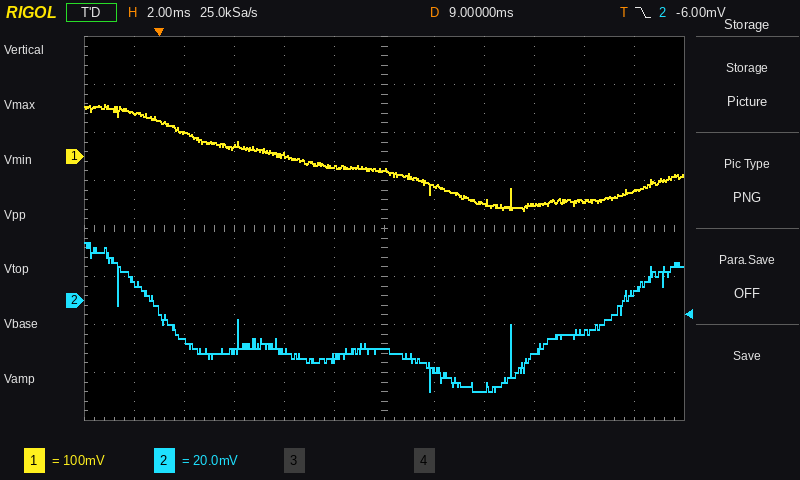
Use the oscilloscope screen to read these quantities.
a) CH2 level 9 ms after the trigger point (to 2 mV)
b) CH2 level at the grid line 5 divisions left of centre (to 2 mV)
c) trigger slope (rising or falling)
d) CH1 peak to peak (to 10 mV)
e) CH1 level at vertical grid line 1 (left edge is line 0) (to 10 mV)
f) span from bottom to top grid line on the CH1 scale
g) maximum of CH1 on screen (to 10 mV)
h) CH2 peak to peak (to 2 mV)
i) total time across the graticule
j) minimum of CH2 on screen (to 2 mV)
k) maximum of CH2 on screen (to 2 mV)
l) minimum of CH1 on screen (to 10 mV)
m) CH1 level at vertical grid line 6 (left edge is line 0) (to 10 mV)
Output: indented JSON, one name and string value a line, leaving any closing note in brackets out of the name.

{
  "CH2 level 9 ms after the trigger point": "-20 mV",
  "CH2 level at the grid line 5 divisions left of centre": "8 mV",
  "trigger slope": "falling",
  "CH1 peak to peak": "220 mV",
  "CH1 level at vertical grid line 1 (left edge is line 0)": "90 mV",
  "span from bottom to top grid line on the CH1 scale": "800 mV",
  "maximum of CH1 on screen": "110 mV",
  "CH2 peak to peak": "62 mV",
  "total time across the graticule": "24 ms",
  "minimum of CH2 on screen": "-38 mV",
  "maximum of CH2 on screen": "24 mV",
  "minimum of CH1 on screen": "-110 mV",
  "CH1 level at vertical grid line 6 (left edge is line 0)": "-30 mV"
}
